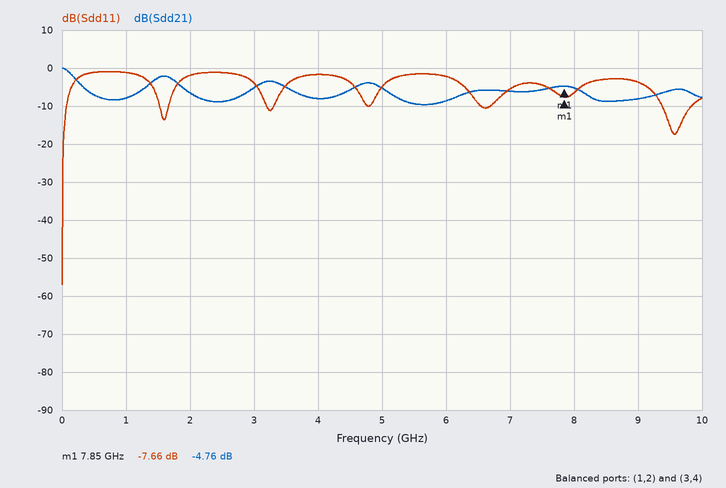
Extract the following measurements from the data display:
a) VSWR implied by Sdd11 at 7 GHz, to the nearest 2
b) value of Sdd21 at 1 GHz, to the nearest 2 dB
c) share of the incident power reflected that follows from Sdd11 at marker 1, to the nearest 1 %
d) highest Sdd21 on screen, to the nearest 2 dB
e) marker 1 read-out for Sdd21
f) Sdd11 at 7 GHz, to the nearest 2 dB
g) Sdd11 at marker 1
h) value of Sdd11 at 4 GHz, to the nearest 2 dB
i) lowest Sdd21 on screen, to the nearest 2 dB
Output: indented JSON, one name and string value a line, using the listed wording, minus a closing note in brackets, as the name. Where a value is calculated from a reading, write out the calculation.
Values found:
{
  "VSWR implied by Sdd11 at 7 GHz, to the nearest 2": "|Γ| = 10^(-6/20) = 0.5012; VSWR = (1 + 0.5012)/(1 − 0.5012) ≈ 3.01, so 4 to the nearest 2",
  "value of Sdd21 at 1 GHz, to the nearest 2 dB": "-8 dB",
  "share of the incident power reflected that follows from Sdd11 at marker 1, to the nearest 1 %": "10^(-7.66/10) ≈ 17 %",
  "highest Sdd21 on screen, to the nearest 2 dB": "0 dB",
  "marker 1 read-out for Sdd21": "-4.76 dB",
  "Sdd11 at 7 GHz, to the nearest 2 dB": "-6 dB",
  "Sdd11 at marker 1": "-7.66 dB",
  "value of Sdd11 at 4 GHz, to the nearest 2 dB": "-2 dB",
  "lowest Sdd21 on screen, to the nearest 2 dB": "-10 dB"
}
